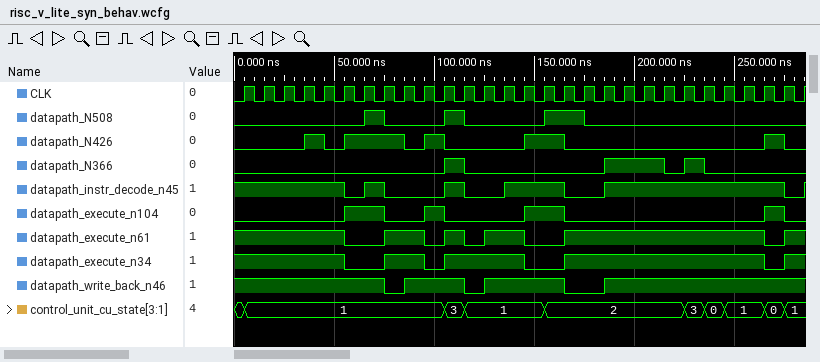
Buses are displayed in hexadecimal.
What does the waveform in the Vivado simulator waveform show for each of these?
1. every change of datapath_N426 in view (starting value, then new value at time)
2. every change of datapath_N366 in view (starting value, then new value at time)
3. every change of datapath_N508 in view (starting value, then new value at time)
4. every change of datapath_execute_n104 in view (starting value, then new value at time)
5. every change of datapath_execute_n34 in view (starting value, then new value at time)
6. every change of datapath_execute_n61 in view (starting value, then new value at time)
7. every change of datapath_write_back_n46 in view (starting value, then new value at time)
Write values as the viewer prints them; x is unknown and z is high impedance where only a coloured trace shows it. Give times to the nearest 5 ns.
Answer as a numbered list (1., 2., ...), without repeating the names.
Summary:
1. 0, 1 at 35 ns, 0 at 45 ns, 1 at 55 ns, 0 at 85 ns, 1 at 95 ns, 0 at 105 ns, 1 at 145 ns, 0 at 165 ns, 1 at 265 ns, 0 at 275 ns
2. 0, 1 at 105 ns, 0 at 115 ns, 1 at 185 ns, 0 at 215 ns, 1 at 225 ns, 0 at 235 ns
3. 0, 1 at 65 ns, 0 at 75 ns, 1 at 105 ns, 0 at 115 ns, 1 at 155 ns, 0 at 175 ns
4. 0, 1 at 55 ns, 0 at 75 ns, 1 at 95 ns, 0 at 105 ns, 1 at 145 ns, 0 at 165 ns, 1 at 265 ns, 0 at 275 ns
5. 1, 0 at 55 ns, 1 at 75 ns, 0 at 95 ns, 1 at 105 ns, 0 at 145 ns, 1 at 165 ns, 0 at 265 ns, 1 at 275 ns
6. 1, 0 at 55 ns, 1 at 75 ns, 0 at 95 ns, 1 at 105 ns, 0 at 115 ns, 1 at 125 ns, 0 at 145 ns, 1 at 165 ns, 0 at 265 ns, 1 at 275 ns
7. 1, 0 at 75 ns, 1 at 85 ns, 0 at 115 ns, 1 at 125 ns, 0 at 165 ns, 1 at 185 ns
